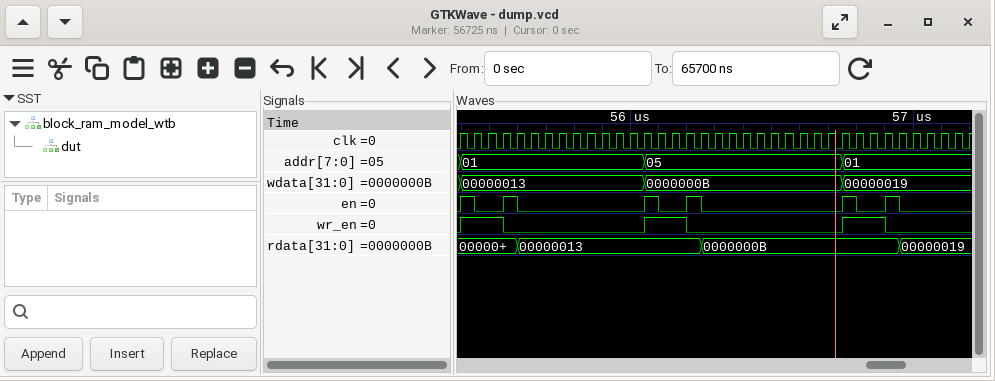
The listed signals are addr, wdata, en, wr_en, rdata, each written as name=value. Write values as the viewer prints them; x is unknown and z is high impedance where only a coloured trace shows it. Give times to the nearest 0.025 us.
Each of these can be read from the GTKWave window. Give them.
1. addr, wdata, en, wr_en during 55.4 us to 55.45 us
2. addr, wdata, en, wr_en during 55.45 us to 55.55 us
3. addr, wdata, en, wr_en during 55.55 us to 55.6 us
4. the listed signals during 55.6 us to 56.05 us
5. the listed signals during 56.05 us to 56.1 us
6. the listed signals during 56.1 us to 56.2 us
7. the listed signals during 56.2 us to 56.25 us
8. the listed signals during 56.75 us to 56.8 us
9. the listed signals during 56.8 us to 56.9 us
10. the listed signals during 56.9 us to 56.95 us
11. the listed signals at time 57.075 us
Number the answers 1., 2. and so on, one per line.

1. addr=01, wdata=00000013, en=1, wr_en=1
2. addr=01, wdata=00000013, en=0, wr_en=1
3. addr=01, wdata=00000013, en=1, wr_en=0
4. addr=01, wdata=00000013, en=0, wr_en=0, rdata=00000013
5. addr=05, wdata=0000000B, en=1, wr_en=1, rdata=00000013
6. addr=05, wdata=0000000B, en=0, wr_en=1, rdata=00000013
7. addr=05, wdata=0000000B, en=1, wr_en=0, rdata=00000013
8. addr=01, wdata=00000019, en=1, wr_en=1, rdata=0000000B
9. addr=01, wdata=00000019, en=0, wr_en=1, rdata=0000000B
10. addr=01, wdata=00000019, en=1, wr_en=0, rdata=0000000B
11. addr=01, wdata=00000019, en=0, wr_en=0, rdata=00000019
